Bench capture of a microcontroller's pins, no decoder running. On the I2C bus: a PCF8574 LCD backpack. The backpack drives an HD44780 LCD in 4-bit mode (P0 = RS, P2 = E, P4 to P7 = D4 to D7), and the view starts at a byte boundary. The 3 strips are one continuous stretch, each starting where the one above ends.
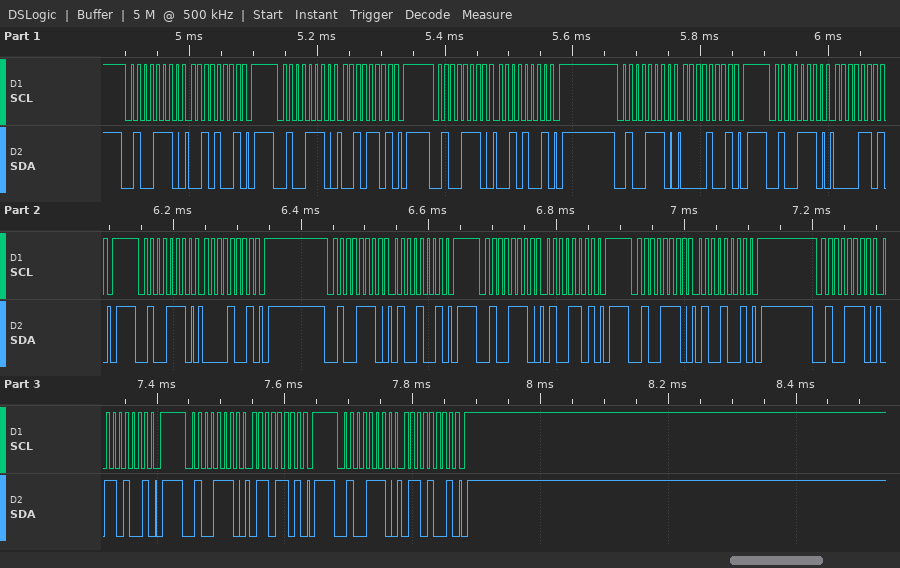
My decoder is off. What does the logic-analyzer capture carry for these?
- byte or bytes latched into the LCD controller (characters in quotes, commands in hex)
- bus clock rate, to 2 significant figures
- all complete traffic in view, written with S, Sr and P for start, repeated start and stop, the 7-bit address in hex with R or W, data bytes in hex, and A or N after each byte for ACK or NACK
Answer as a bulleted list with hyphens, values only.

- ' ' 'F'
- 100 kHz
- S 27W A 29 A P S 27W A 2D A P S 27W A 29 A P S 27W A 09 A P S 27W A 0D A P S 27W A 09 A P S 27W A 49 A P S 27W A 4D A P S 27W A 49 A P S 27W A 69 A P S 27W A 6D A P S 27W A 69 A P
